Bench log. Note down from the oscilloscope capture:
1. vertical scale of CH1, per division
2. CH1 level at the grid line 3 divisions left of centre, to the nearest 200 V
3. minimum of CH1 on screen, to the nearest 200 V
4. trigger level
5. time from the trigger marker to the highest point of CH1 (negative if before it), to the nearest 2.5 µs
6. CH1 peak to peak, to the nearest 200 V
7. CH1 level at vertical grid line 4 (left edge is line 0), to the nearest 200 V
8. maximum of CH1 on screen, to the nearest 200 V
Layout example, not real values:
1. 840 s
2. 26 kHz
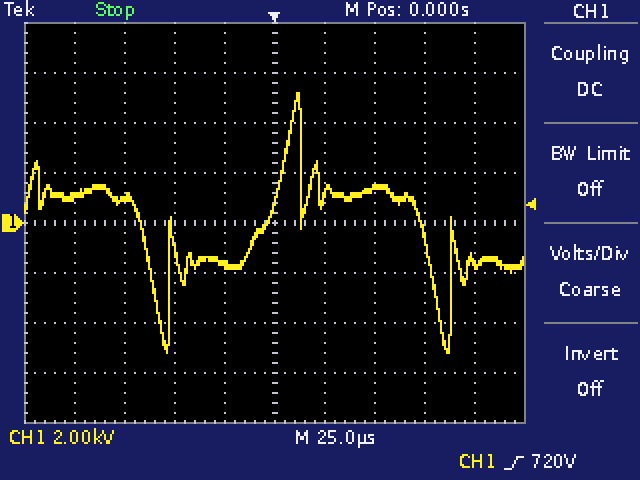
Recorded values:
1. 2 kV
2. 1.0 kV
3. -5.2 kV
4. 720 V
5. +12.5 µs
6. 10.4 kV
7. -1.6 kV
8. 5.2 kV
